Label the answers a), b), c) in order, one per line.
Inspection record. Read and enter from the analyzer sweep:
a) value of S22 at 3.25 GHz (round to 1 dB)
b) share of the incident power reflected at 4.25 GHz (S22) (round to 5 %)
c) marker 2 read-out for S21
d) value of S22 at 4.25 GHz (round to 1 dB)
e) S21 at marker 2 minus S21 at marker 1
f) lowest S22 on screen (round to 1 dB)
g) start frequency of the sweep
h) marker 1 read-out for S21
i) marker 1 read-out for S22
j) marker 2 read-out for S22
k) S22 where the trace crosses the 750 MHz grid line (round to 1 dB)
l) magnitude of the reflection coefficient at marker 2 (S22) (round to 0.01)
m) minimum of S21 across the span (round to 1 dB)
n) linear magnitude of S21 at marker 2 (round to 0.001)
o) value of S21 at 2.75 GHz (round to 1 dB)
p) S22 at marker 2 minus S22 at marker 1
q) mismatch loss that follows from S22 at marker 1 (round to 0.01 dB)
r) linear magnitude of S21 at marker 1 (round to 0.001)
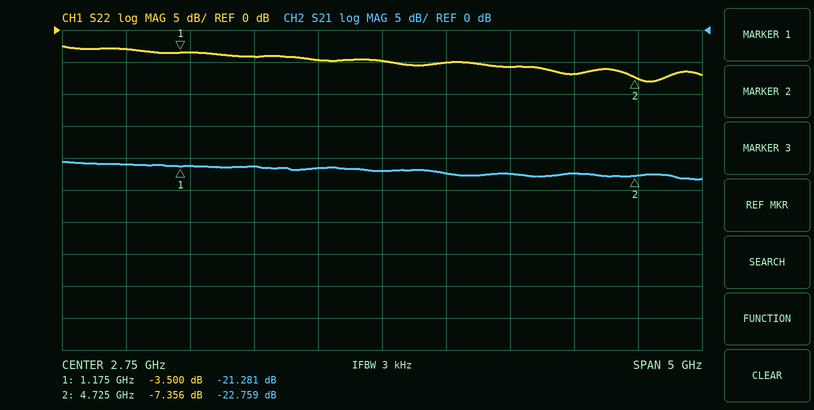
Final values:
a) -5 dB
b) 20 %
c) -22.759 dB
d) -7 dB
e) -1.478 dB
f) -8 dB
g) 250 MHz
h) -21.281 dB
i) -3.500 dB
j) -7.356 dB
k) -3 dB
l) 0.43
m) -23 dB
n) 0.073
o) -22 dB
p) -3.856 dB
q) 2.57 dB
r) 0.086
